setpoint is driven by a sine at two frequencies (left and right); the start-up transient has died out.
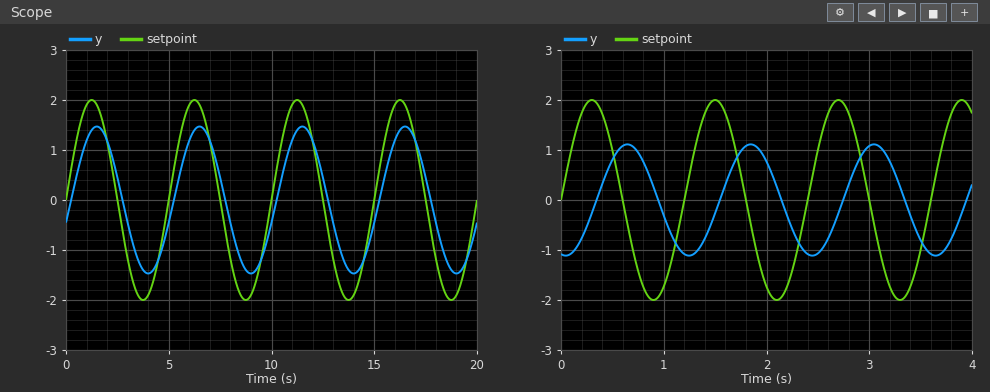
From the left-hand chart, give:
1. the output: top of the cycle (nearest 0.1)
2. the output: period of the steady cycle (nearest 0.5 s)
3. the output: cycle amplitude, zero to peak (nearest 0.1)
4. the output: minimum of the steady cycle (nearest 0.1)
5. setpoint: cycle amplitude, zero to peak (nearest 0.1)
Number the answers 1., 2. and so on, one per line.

1. 1.5
2. 5.0 s
3. 1.5
4. -1.5
5. 2.0
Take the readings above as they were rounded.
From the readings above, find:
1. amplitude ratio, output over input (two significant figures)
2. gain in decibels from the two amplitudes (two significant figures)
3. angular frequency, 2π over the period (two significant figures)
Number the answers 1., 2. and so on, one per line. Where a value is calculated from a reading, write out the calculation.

1. 1.5 / 2 = 0.75
2. 20 log10(1.5 / 2) = -2.5 dB
3. 2π / 5 = 1.3 rad/s
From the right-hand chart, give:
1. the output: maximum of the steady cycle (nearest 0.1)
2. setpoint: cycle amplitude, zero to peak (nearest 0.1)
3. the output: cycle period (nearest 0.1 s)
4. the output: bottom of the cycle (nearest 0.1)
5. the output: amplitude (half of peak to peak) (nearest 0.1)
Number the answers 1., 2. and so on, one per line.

1. 1.1
2. 2.0
3. 1.2 s
4. -1.1
5. 1.1
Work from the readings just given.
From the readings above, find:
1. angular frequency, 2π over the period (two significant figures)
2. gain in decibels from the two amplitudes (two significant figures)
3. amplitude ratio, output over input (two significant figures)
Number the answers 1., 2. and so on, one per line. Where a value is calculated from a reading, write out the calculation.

1. 2π / 1.2 = 5.2 rad/s
2. 20 log10(1.1 / 2) = -5.2 dB
3. 1.1 / 2 = 0.55
